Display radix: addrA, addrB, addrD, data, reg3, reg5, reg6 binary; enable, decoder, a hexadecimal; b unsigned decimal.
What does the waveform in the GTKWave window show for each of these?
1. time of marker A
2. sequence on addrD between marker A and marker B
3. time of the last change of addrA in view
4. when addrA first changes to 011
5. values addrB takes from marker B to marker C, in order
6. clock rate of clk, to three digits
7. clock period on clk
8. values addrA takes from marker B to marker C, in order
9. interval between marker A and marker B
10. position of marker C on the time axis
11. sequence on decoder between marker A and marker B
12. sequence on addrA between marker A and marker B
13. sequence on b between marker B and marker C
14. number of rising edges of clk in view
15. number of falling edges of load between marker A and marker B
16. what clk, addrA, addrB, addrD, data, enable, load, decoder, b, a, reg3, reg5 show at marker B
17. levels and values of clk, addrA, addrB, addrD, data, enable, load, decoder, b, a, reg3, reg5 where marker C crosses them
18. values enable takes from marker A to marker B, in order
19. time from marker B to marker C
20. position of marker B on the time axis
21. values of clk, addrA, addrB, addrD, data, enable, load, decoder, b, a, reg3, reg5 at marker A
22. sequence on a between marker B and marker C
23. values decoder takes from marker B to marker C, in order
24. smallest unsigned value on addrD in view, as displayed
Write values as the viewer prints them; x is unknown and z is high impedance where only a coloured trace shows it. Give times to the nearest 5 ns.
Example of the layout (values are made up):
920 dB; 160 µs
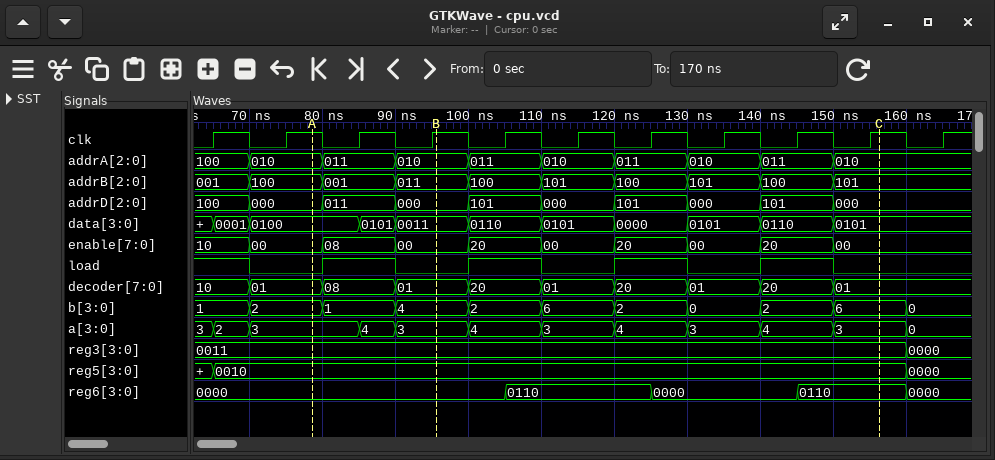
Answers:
80 ns; 000, 011, 000; 150 ns; 80 ns; 011, 100, 101, 100, 101, 100, 101; 100 MHz; 10 ns; 010, 011, 010, 011, 010, 011, 010; 15 ns; 155 ns; 01, 08, 01; 010, 011, 010; 4, 2, 6, 2, 0, 2, 6; 11; 1; clk=1, addrA=010, addrB=011, addrD=000, data=0011, enable=00, load=0, decoder=01, b=4, a=3, reg3=0011, reg5=0010; clk=1, addrA=010, addrB=101, addrD=000, data=0101, enable=00, load=0, decoder=01, b=6, a=3, reg3=0011, reg5=0010; 00, 08, 00; 60 ns; 95 ns; clk=1, addrA=010, addrB=100, addrD=000, data=0100, enable=00, load=0, decoder=01, b=2, a=3, reg3=0011, reg5=0010; 3, 4, 3, 4, 3, 4, 3; 01, 20, 01, 20, 01, 20, 01; 000
